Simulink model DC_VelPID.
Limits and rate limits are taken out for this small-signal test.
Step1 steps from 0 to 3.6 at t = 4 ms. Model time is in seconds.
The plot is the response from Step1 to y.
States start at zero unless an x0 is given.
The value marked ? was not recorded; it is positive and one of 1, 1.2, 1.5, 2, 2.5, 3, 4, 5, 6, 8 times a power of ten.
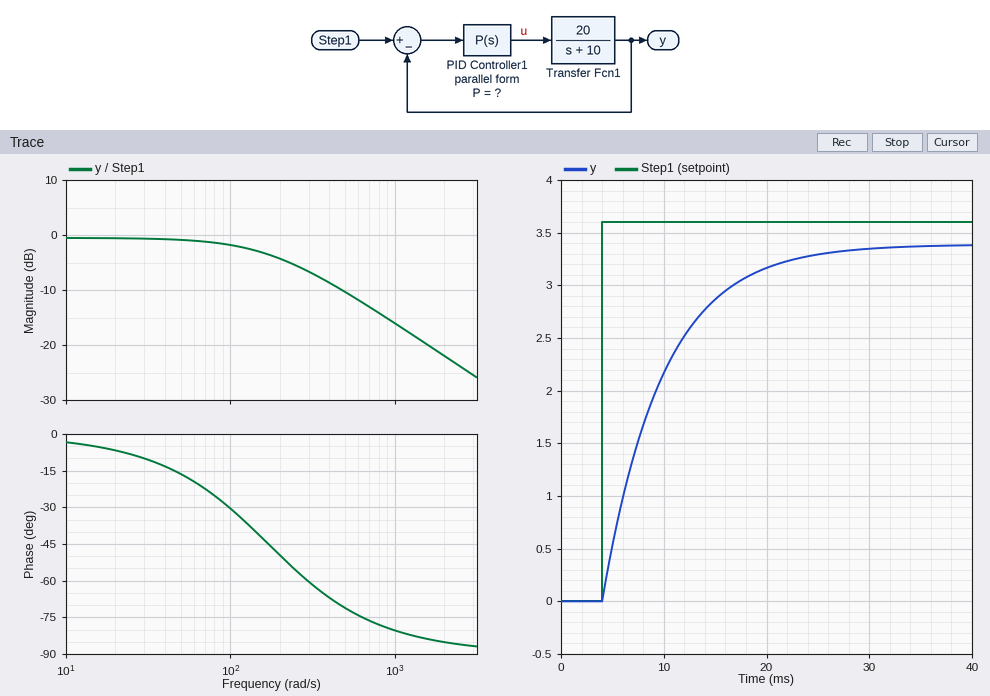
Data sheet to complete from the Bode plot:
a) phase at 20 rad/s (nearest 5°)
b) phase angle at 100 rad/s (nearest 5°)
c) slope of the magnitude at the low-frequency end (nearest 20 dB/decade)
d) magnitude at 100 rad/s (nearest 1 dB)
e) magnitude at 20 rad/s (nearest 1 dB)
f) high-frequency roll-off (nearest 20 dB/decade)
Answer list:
-5°
-30°
0 dB/decade
-2 dB
-1 dB
-20 dB/decade
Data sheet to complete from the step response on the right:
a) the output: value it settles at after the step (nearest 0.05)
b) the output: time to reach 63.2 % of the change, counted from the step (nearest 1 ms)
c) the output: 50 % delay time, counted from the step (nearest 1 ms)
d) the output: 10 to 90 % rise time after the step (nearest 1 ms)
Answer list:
3.40
6 ms
4 ms
13 ms
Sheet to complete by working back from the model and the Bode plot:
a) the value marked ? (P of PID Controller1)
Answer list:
8
